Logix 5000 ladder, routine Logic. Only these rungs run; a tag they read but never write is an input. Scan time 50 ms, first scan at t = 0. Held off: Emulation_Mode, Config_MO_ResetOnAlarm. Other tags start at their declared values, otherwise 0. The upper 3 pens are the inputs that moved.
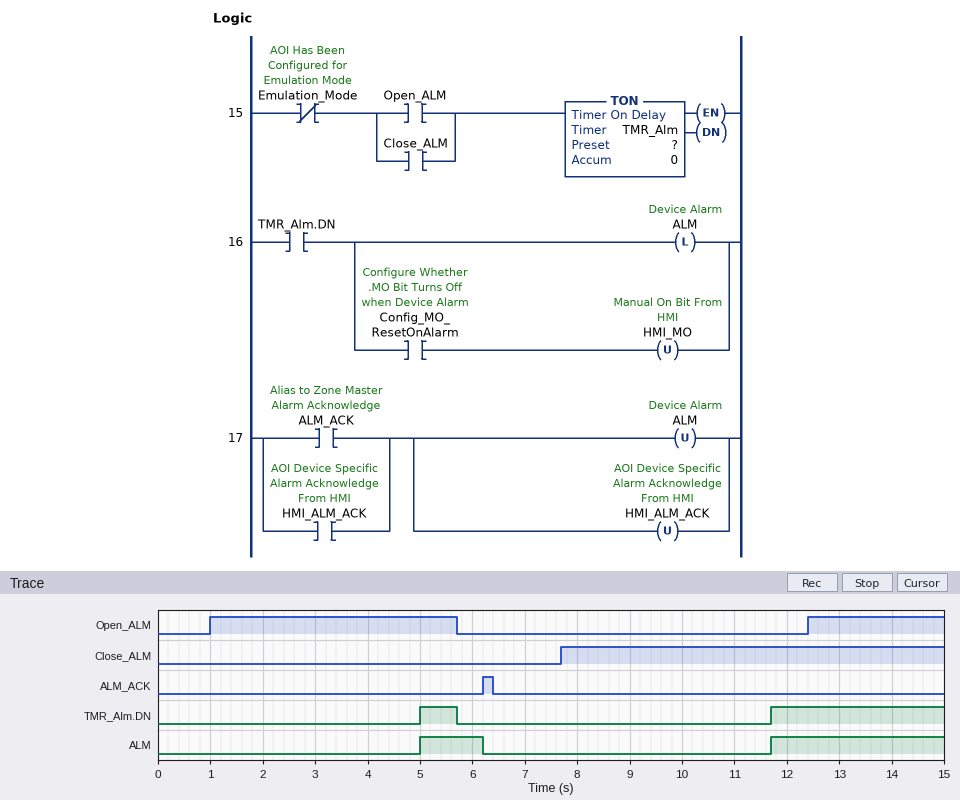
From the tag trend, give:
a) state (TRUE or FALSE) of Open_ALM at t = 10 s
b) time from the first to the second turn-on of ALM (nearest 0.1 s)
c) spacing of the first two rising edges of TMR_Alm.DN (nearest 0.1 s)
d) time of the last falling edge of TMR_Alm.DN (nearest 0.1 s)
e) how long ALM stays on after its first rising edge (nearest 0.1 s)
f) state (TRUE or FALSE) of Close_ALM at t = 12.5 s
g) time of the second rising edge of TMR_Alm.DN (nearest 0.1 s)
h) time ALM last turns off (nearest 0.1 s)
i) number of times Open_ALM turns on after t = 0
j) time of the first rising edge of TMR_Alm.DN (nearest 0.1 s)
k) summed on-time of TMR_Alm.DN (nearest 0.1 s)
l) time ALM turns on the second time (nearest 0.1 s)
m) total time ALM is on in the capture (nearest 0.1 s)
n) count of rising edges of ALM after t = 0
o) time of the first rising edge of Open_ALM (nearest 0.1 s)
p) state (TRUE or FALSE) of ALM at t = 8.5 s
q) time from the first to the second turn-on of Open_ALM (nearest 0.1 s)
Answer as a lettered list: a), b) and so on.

a) FALSE
b) 6.7 s
c) 6.7 s
d) 5.7 s
e) 1.2 s
f) TRUE
g) 11.7 s
h) 6.2 s
i) 2
j) 5.0 s
k) 4.0 s
l) 11.7 s
m) 4.5 s
n) 2
o) 1.0 s
p) FALSE
q) 11.4 s
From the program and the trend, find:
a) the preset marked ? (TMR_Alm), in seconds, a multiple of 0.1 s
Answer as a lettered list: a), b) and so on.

a) 4.0 s
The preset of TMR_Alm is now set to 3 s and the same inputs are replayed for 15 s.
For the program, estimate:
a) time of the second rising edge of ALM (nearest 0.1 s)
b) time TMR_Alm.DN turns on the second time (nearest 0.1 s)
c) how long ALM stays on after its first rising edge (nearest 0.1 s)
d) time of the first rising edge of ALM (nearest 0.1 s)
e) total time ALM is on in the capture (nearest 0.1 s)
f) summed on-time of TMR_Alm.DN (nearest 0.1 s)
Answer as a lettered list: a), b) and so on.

a) 10.7 s
b) 10.7 s
c) 2.2 s
d) 4.0 s
e) 6.5 s
f) 6.0 s
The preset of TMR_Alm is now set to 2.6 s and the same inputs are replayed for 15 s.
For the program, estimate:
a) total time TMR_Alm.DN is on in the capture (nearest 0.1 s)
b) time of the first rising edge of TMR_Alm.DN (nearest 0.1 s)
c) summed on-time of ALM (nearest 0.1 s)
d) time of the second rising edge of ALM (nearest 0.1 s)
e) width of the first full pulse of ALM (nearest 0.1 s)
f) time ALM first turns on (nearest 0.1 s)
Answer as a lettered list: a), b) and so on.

a) 6.8 s
b) 3.6 s
c) 7.3 s
d) 10.3 s
e) 2.6 s
f) 3.6 s
